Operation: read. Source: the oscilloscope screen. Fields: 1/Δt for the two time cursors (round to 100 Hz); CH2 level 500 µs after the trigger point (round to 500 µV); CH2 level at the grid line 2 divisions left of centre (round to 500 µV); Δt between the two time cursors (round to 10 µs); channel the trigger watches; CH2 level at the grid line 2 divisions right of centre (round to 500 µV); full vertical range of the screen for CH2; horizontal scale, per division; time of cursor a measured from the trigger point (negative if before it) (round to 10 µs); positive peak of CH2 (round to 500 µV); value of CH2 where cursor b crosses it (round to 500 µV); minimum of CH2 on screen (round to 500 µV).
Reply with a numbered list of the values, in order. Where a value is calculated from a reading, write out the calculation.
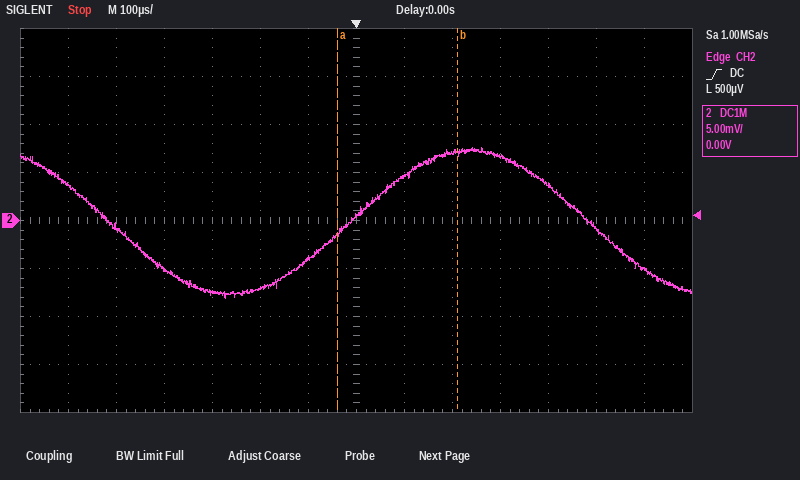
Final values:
1. 1 / 250 µs ≈ 4.0 kHz
2. -1.0 mV
3. -7.0 mV
4. 250 µs
5. CH2
6. 7.0 mV
7. 40 mV
8. 100 µs
9. -40 µs
10. 7.5 mV
11. 7.0 mV
12. -8.0 mV
